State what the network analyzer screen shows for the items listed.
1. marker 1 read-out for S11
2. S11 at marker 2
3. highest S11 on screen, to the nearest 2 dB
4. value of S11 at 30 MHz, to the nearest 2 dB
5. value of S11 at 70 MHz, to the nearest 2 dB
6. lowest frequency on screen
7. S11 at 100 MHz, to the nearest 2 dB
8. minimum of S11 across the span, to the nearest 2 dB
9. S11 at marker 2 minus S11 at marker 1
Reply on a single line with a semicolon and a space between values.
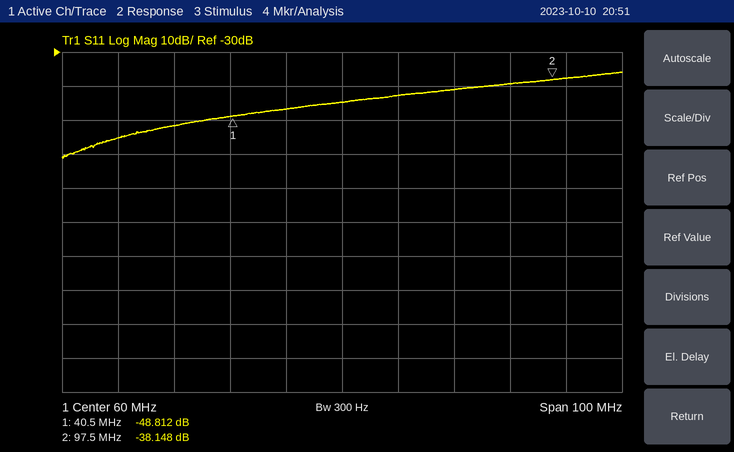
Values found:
-48.812 dB; -38.148 dB; -36 dB; -52 dB; -42 dB; 10 MHz; -38 dB; -62 dB; 10.664 dB
